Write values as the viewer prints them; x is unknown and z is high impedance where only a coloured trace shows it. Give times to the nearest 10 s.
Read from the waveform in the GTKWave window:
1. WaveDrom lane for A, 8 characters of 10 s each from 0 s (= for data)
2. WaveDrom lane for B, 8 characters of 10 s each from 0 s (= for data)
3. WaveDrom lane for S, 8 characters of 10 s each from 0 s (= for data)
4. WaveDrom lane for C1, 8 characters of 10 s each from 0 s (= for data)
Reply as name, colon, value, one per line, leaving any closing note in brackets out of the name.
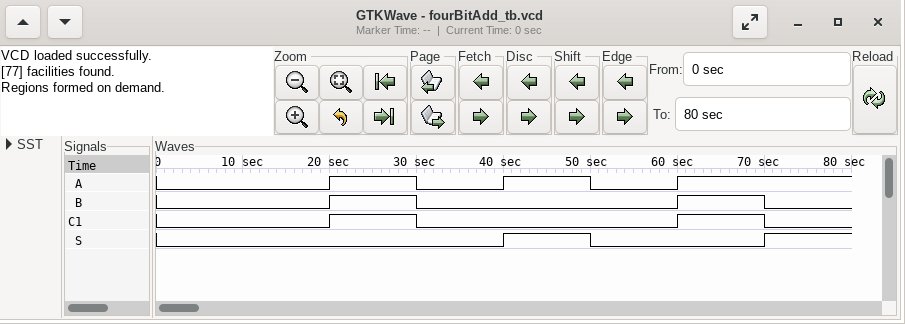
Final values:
WaveDrom lane for A, 8 characters of 10 s each from 0 s: {name: 'A', wave: '0.10101.'}
WaveDrom lane for B, 8 characters of 10 s each from 0 s: {name: 'B', wave: '0.10..10'}
WaveDrom lane for S, 8 characters of 10 s each from 0 s: {name: 'S', wave: '0...10.1'}
WaveDrom lane for C1, 8 characters of 10 s each from 0 s: {name: 'C1', wave: '0.10..10'}
